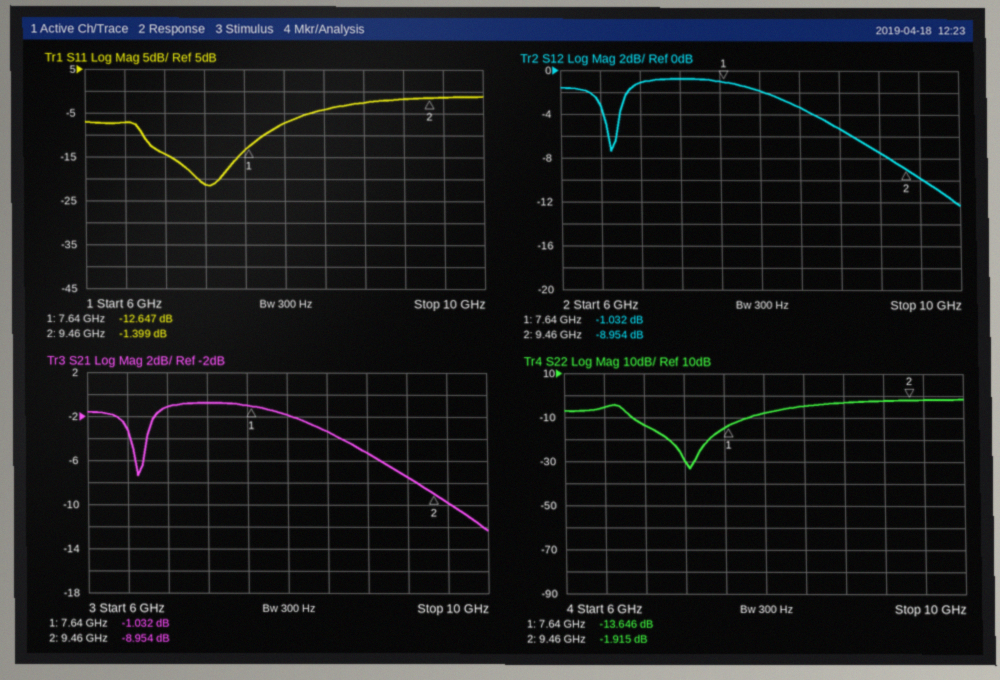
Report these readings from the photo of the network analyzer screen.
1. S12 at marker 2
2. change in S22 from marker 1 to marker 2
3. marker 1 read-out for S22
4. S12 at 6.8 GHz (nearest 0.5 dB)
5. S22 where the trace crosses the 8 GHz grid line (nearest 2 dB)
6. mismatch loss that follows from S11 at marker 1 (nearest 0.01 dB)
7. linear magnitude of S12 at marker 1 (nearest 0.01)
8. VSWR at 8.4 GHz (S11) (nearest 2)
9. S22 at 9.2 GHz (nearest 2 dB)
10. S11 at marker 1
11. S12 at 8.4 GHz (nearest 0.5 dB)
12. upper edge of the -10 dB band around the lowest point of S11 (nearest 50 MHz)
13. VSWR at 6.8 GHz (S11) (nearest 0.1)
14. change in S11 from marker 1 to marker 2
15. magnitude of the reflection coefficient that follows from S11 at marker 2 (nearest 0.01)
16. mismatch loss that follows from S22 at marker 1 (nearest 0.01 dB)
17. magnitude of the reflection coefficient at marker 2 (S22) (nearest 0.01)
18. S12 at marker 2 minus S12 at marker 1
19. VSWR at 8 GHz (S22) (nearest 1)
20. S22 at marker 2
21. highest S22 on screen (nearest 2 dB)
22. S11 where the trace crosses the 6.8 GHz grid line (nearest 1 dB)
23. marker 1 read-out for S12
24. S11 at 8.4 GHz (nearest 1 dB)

-8.954 dB
11.731 dB
-13.646 dB
-1.0 dB
-8 dB
0.24 dB
0.89
4
-2 dB
-12.647 dB
-3.5 dB
7.80 GHz
1.5
11.248 dB
0.85
0.19 dB
0.80
-7.922 dB
2
-1.915 dB
-2 dB
-14 dB
-1.032 dB
-4 dB
